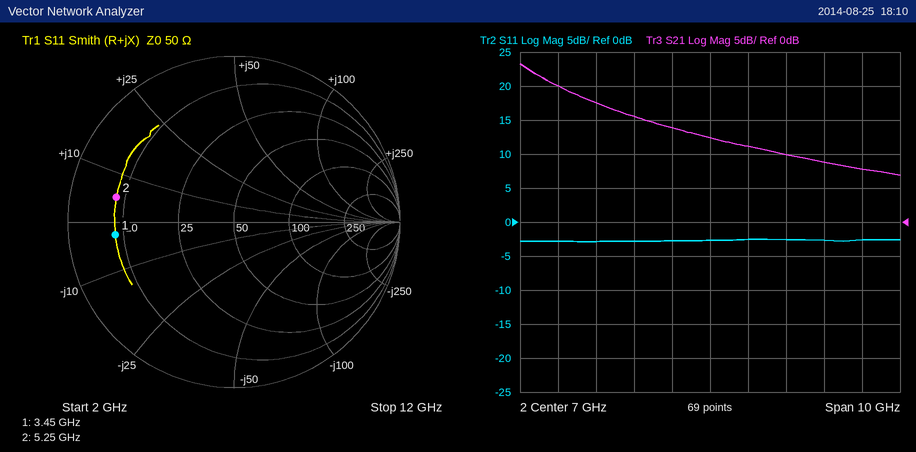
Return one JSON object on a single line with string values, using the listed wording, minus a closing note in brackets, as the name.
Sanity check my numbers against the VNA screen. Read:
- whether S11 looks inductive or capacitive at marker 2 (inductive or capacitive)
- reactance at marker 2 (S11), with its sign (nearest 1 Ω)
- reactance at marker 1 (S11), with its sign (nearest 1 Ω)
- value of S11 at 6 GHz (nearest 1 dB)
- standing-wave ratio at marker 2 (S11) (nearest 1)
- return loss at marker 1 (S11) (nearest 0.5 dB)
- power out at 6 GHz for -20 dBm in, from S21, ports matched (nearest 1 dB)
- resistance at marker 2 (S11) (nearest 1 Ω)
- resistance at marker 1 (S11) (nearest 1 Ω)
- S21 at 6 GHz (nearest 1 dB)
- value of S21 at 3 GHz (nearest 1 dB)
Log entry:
{"whether S11 looks inductive or capacitive at marker 2": "inductive", "reactance at marker 2 (S11), with its sign": "+5 Ω", "reactance at marker 1 (S11), with its sign": "-3 Ω", "value of S11 at 6 GHz": "-3 dB", "standing-wave ratio at marker 2 (S11)": "6", "return loss at marker 1 (S11)": "3.0 dB", "power out at 6 GHz for -20 dBm in, from S21, ports matched": "-6 dBm", "resistance at marker 2 (S11)": "8 Ω", "resistance at marker 1 (S11)": "8 Ω", "S21 at 6 GHz": "14 dB", "value of S21 at 3 GHz": "20 dB"}
